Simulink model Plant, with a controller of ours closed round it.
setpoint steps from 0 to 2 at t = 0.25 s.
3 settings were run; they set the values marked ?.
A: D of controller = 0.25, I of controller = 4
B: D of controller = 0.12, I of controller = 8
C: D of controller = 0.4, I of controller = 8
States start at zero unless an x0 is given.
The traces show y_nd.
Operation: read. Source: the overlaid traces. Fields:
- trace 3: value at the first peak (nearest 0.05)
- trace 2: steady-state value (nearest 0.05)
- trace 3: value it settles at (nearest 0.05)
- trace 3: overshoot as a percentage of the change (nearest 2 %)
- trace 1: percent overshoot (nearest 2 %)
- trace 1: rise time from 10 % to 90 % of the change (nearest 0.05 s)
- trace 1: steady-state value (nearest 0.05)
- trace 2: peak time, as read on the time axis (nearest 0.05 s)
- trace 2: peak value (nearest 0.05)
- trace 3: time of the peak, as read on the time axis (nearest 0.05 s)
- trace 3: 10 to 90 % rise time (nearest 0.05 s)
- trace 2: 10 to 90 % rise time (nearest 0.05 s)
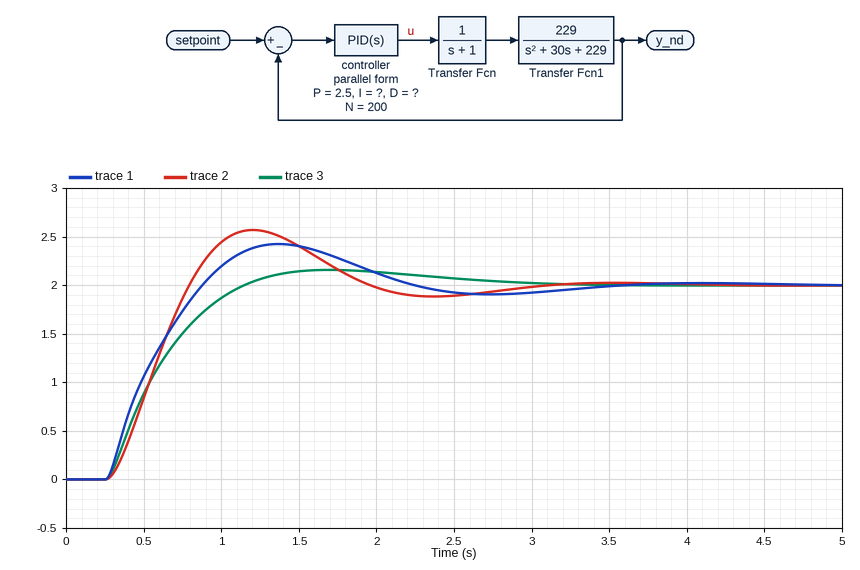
2.15
2.00
2.00
8 %
22 %
0.45 s
2.00
1.20 s
2.55
1.70 s
0.60 s
0.40 s
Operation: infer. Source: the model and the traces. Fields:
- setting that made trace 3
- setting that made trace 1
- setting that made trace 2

A
C
B
